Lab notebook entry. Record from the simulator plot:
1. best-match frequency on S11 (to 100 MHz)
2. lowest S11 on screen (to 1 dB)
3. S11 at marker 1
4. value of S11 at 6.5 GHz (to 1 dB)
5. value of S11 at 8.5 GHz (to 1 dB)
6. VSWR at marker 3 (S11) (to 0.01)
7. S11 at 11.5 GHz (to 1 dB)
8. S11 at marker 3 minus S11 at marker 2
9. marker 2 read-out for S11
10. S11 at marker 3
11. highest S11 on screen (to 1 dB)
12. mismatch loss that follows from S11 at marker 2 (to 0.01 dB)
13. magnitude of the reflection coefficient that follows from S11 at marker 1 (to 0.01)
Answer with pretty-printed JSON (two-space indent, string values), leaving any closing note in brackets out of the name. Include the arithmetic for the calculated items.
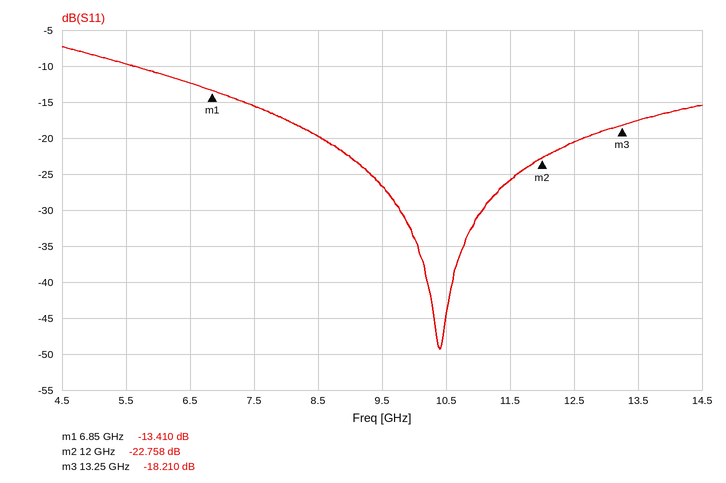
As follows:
{
  "best-match frequency on S11": "10.4 GHz",
  "lowest S11 on screen": "-49 dB",
  "S11 at marker 1": "-13.410 dB",
  "value of S11 at 6.5 GHz": "-12 dB",
  "value of S11 at 8.5 GHz": "-20 dB",
  "VSWR at marker 3 (S11)": "(1 + 0.1229)/(1 − 0.1229) ≈ 1.28",
  "S11 at 11.5 GHz": "-26 dB",
  "S11 at marker 3 minus S11 at marker 2": "-18.21 − (-22.758) = 4.548 dB",
  "marker 2 read-out for S11": "-22.758 dB",
  "S11 at marker 3": "-18.210 dB",
  "highest S11 on screen": "-7 dB",
  "mismatch loss that follows from S11 at marker 2": "−10 log10(1 − 10^(-22.758/10)) ≈ 0.02 dB",
  "magnitude of the reflection coefficient that follows from S11 at marker 1": "10^(-13.41/20) ≈ 0.21"
}
